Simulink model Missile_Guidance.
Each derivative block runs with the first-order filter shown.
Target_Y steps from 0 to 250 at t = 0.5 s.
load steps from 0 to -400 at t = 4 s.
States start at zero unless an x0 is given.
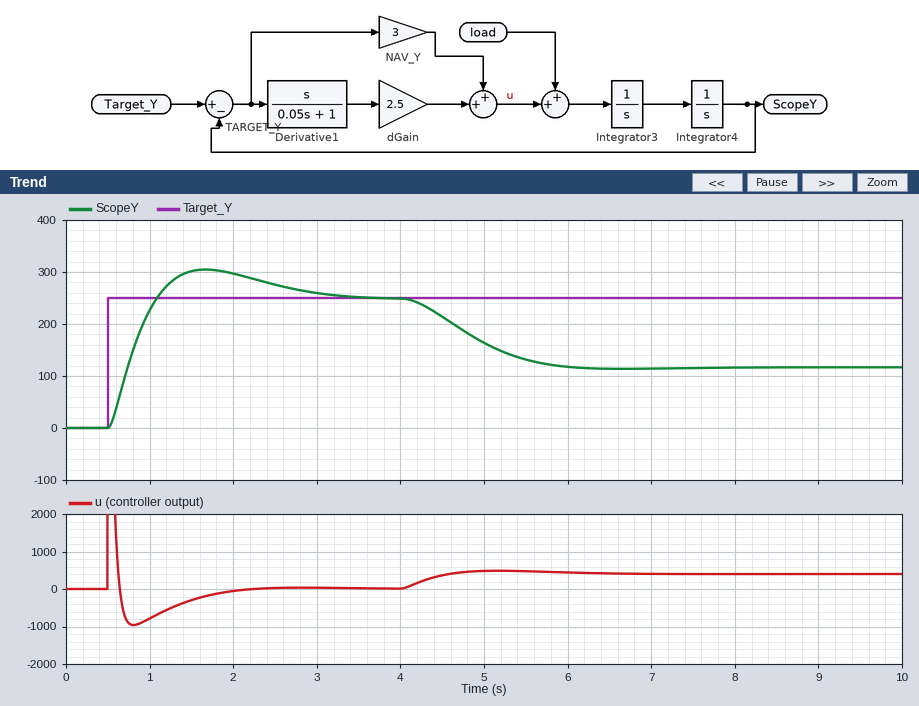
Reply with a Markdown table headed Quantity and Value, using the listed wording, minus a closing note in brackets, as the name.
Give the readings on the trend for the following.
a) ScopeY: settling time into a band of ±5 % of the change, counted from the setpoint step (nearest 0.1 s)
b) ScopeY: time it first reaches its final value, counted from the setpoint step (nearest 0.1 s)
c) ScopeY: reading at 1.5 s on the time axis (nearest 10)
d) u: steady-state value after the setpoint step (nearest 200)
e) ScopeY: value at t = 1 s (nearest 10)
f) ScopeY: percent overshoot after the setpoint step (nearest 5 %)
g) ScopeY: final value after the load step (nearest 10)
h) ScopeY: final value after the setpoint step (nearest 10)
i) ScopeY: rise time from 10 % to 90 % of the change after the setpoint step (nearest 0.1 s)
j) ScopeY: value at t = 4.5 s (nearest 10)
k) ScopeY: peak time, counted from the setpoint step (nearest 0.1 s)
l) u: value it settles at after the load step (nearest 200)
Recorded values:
| Quantity | Value |
|---|---|
| ScopeY: settling time into a band of ±5 % of the change, counted from the setpoint step | 2.4 s |
| ScopeY: time it first reaches its final value, counted from the setpoint step | 0.6 s |
| ScopeY: reading at 1.5 s on the time axis | 300 |
| u: steady-state value after the setpoint step | 0 |
| ScopeY: value at t = 1 s | 230 |
| ScopeY: percent overshoot after the setpoint step | 20 % |
| ScopeY: final value after the load step | 120 |
| ScopeY: final value after the setpoint step | 250 |
| ScopeY: rise time from 10 % to 90 % of the change after the setpoint step | 0.4 s |
| ScopeY: value at t = 4.5 s | 210 |
| ScopeY: peak time, counted from the setpoint step | 1.2 s |
| u: value it settles at after the load step | 400 |
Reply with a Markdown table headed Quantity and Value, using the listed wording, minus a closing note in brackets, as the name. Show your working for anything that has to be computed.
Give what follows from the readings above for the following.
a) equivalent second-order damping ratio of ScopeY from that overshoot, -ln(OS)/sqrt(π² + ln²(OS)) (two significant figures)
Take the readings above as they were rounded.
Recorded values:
| Quantity | Value |
|---|---|
| equivalent second-order damping ratio of ScopeY from that overshoot, -ln(OS)/sqrt(π² + ln²(OS)) | ln(0.2) = -1.609; 1.609 / sqrt(9.870 + 2.590) = 0.46 |
